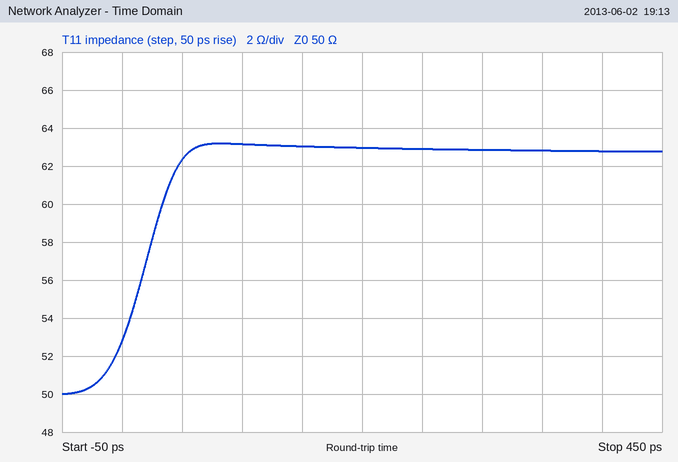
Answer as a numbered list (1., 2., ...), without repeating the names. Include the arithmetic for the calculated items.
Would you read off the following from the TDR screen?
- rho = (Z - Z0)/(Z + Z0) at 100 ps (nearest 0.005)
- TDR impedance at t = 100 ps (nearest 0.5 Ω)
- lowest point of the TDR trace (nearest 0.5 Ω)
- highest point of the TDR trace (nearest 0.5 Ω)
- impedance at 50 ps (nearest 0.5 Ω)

1. (63 − 50)/(63 + 50) ≈ +0.115
2. 63.0 Ω
3. 50.0 Ω
4. 63.0 Ω
5. 62.5 Ω
